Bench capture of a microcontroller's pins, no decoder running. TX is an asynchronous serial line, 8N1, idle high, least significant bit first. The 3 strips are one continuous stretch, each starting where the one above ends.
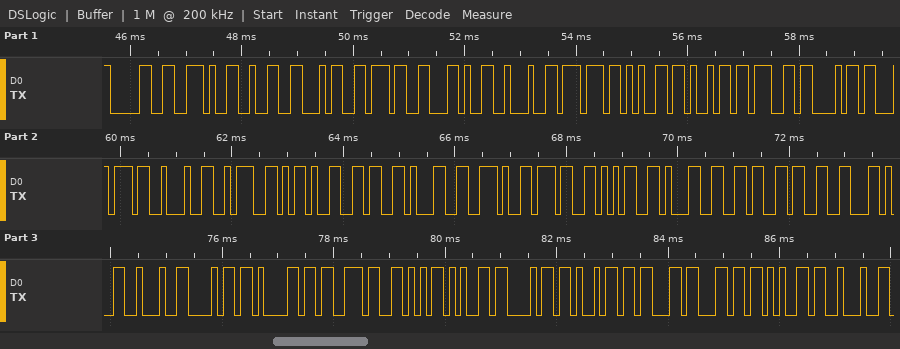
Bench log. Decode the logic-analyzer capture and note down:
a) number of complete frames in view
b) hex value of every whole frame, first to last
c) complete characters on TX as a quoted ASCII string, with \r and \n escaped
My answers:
37
30 2E 32 34 37 2C 22 77 65 69 67 68 74 22 3A 2D 36 31 2E 37 35 31 36 33 2C 22 68 61 73 56 65 68 69 63 6C 65 22
"0.247,\"weight\":-61.75163,\"hasVehicle\""
